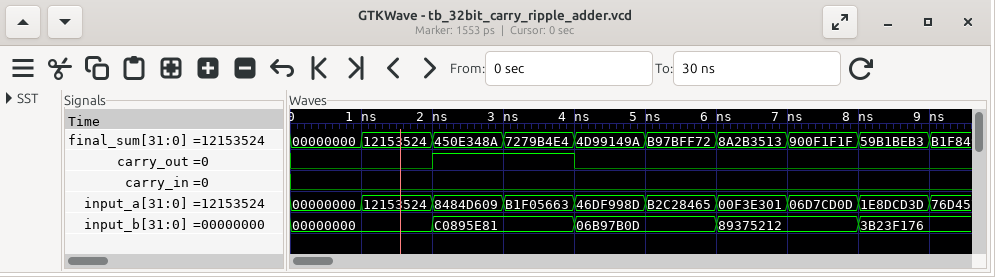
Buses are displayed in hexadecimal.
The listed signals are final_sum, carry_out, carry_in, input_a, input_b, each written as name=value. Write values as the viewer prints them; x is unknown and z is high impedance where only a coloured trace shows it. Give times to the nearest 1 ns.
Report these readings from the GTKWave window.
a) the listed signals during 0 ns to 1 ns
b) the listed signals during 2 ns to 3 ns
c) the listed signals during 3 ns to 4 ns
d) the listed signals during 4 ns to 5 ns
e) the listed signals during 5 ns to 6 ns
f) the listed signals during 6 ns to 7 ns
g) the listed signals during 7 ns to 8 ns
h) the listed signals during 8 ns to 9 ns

final_sum=00000000, carry_out=0, carry_in=0, input_a=00000000, input_b=00000000
final_sum=450E348A, carry_out=1, carry_in=0, input_a=8484D609, input_b=C0895E81
final_sum=7279B4E4, carry_out=1, carry_in=0, input_a=B1F05663, input_b=C0895E81
final_sum=4D99149A, carry_out=0, carry_in=0, input_a=46DF998D, input_b=06B97B0D
final_sum=B97BFF72, carry_out=0, carry_in=0, input_a=B2C28465, input_b=06B97B0D
final_sum=8A2B3513, carry_out=0, carry_in=0, input_a=00F3E301, input_b=89375212
final_sum=900F1F1F, carry_out=0, carry_in=0, input_a=06D7CD0D, input_b=89375212
final_sum=59B1BEB3, carry_out=0, carry_in=0, input_a=1E8DCD3D, input_b=3B23F176
